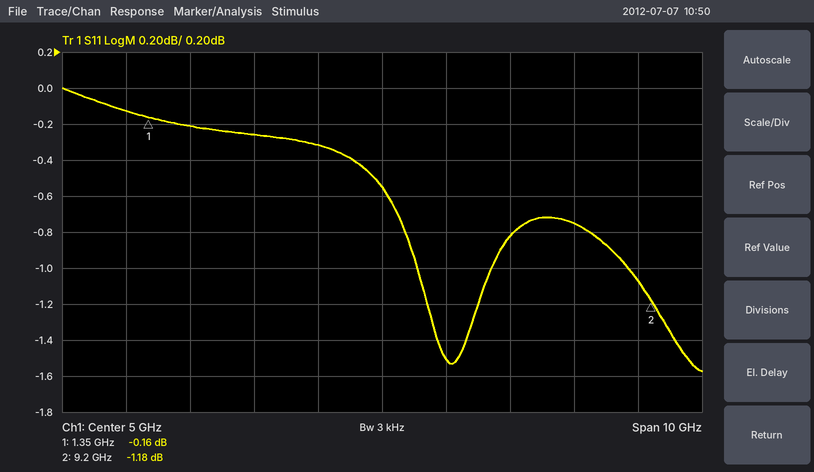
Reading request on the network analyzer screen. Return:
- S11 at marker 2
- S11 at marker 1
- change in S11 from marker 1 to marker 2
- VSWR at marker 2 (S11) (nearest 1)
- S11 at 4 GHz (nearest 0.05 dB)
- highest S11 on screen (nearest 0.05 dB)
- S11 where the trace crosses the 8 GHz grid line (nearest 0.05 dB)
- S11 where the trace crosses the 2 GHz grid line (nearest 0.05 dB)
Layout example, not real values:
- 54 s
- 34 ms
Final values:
- -1.18 dB
- -0.16 dB
- -1.02 dB
- 15
- -0.30 dB
- 0.00 dB
- -0.75 dB
- -0.20 dB
